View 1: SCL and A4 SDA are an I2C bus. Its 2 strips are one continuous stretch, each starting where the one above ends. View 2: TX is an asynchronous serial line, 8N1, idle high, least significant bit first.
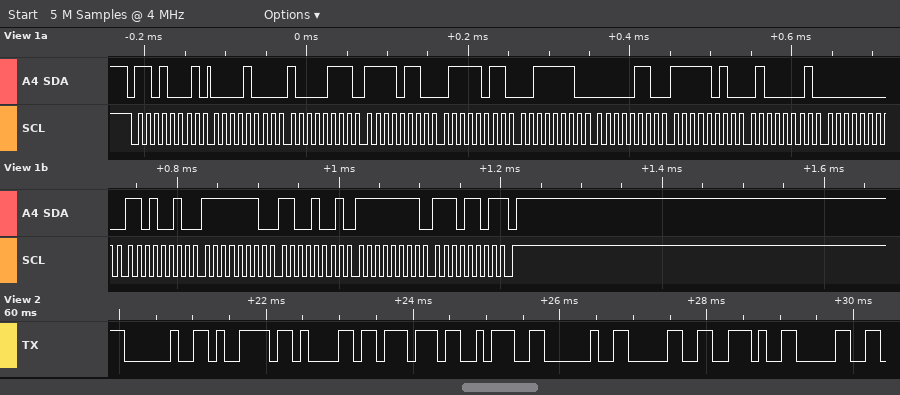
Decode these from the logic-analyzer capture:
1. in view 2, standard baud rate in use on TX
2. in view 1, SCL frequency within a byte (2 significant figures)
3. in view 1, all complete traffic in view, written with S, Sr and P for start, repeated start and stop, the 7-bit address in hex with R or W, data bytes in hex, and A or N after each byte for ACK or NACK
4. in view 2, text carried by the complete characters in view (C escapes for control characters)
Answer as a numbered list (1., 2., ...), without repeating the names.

1. 9600 baud
2. 100 kHz
3. S 68R A 08 A 87 A F6 A 7B A 3E A 06 A FA A 41 A 00 A D2 A FE A C9 A FF A ED N P
4. " yaw: 0.0"
